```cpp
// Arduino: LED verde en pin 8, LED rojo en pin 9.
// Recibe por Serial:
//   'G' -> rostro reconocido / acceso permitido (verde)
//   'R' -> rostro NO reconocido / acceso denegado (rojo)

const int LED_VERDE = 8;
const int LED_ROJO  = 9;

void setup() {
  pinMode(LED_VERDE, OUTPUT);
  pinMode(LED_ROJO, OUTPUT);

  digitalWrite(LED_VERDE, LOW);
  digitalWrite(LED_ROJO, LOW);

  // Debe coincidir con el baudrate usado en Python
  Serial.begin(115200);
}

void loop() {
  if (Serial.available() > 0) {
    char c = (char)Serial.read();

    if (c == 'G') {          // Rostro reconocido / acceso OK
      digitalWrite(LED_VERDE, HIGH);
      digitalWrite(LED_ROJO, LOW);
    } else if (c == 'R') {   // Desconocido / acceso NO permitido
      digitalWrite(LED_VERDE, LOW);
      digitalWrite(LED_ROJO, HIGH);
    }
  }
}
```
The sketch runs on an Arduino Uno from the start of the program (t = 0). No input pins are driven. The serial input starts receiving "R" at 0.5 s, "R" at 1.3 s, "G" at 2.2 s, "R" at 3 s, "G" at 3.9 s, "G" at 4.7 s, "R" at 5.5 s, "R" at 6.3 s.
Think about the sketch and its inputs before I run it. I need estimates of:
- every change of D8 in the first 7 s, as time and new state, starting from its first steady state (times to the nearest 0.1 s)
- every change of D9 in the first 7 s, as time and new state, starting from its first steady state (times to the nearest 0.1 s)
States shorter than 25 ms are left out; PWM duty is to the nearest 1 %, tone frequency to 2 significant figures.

0 s low; 2.2 s high; 3 s low; 3.9 s high; 5.5 s low
0 s low; 0.5 s high; 2.2 s low; 3 s high; 3.9 s low; 5.5 s high
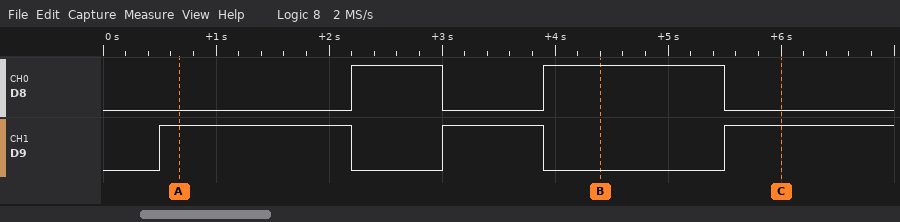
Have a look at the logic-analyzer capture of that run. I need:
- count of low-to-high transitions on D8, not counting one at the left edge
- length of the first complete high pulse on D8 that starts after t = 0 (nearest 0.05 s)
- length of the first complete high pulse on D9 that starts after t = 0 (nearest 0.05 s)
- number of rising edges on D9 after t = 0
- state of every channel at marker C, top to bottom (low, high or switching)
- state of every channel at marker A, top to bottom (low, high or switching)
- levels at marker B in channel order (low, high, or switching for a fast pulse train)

2
0.80 s
1.70 s
3
D8 low, D9 high
D8 low, D9 high
D8 high, D9 low
